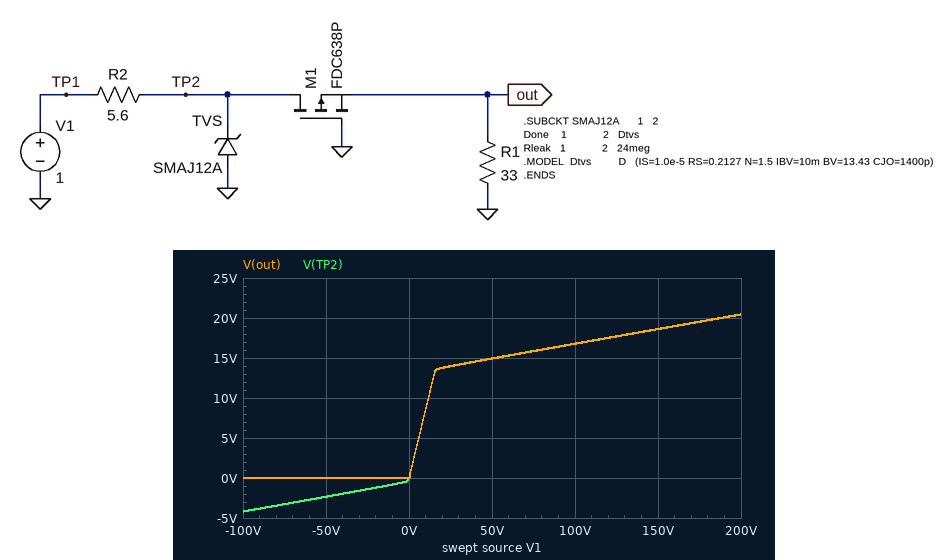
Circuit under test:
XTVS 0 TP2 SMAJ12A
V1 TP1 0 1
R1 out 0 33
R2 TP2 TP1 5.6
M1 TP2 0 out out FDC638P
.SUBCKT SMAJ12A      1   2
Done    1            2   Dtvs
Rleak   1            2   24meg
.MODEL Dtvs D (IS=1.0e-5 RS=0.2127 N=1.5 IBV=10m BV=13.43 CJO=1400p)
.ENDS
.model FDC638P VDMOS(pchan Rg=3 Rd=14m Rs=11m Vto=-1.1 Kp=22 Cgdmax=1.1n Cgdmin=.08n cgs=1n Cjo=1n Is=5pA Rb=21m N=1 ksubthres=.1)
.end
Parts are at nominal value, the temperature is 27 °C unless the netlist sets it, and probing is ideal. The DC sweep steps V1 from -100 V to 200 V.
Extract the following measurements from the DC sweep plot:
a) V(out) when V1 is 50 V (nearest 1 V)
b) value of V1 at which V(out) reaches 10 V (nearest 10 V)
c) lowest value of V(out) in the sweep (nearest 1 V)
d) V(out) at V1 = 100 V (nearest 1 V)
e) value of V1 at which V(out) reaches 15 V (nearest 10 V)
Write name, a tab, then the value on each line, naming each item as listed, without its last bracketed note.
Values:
V(out) when V1 is 50 V	15 V
value of V1 at which V(out) reaches 10 V	10 V
lowest value of V(out) in the sweep	0 V
V(out) at V1 = 100 V	17 V
value of V1 at which V(out) reaches 15 V	50 V
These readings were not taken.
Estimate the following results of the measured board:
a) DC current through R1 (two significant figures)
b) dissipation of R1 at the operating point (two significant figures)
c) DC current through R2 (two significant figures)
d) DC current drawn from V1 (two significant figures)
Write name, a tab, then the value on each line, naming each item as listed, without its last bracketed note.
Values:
DC current through R1	12 mA
dissipation of R1 at the operating point	4.5 mW
DC current through R2	12 mA
DC current drawn from V1	12 mA
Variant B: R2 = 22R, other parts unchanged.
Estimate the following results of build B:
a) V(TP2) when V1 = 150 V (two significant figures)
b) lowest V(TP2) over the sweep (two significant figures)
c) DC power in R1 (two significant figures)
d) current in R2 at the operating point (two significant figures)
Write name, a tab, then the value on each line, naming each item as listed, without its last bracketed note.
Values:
V(TP2) when V1 = 150 V	15 V
lowest V(TP2) over the sweep	-1.5 V
DC power in R1	2.2 mW
current in R2 at the operating point	8.2 mA
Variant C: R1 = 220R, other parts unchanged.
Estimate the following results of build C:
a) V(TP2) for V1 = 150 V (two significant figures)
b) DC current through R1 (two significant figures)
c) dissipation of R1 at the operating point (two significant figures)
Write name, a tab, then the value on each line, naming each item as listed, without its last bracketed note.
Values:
V(TP2) for V1 = 150 V	19 V
DC current through R1	4.4 mA
dissipation of R1 at the operating point	4.2 mW
